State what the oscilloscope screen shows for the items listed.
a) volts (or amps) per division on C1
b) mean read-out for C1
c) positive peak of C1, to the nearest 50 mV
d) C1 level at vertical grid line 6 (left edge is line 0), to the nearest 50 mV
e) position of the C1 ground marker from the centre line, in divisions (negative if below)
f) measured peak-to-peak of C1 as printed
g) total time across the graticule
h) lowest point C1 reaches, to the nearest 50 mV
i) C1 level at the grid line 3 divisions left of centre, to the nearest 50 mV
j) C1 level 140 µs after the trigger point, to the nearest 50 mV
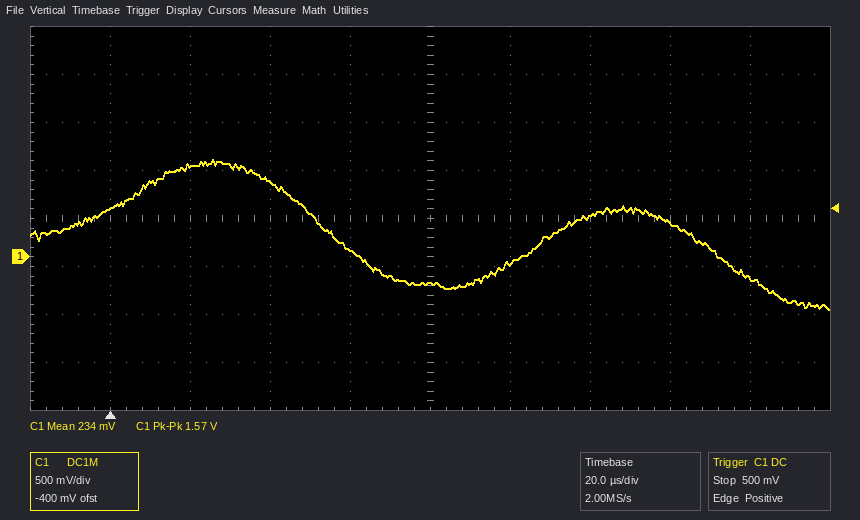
500 mV
234 mV
1.00 V
-50 mV
-0.8 div
1.57 V
200 µs
-550 mV
950 mV
350 mV
